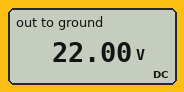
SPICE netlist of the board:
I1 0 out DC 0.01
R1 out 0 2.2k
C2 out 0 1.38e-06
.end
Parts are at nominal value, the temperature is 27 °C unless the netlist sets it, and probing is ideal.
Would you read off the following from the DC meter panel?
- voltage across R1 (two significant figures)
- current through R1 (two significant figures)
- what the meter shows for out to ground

22 V
10 mA
22.00 V
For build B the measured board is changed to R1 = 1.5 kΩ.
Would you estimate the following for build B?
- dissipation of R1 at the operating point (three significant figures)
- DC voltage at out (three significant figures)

150 mW
15.0 V
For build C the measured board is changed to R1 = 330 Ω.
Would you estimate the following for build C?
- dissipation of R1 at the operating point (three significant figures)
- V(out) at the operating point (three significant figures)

33.0 mW
3.30 V
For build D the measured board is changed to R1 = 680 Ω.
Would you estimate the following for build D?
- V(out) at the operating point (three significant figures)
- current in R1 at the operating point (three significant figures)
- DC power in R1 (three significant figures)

6.80 V
10.0 mA
68.0 mW
